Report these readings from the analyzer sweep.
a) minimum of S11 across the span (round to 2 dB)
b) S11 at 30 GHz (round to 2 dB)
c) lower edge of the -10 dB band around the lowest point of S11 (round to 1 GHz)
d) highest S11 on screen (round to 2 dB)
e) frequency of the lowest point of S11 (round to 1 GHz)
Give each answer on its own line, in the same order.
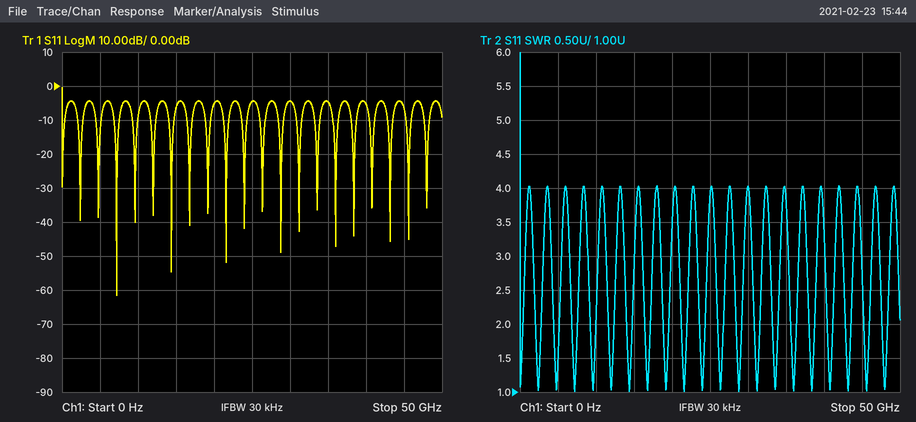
-62 dB
-4 dB
7 GHz
0 dB
7 GHz
